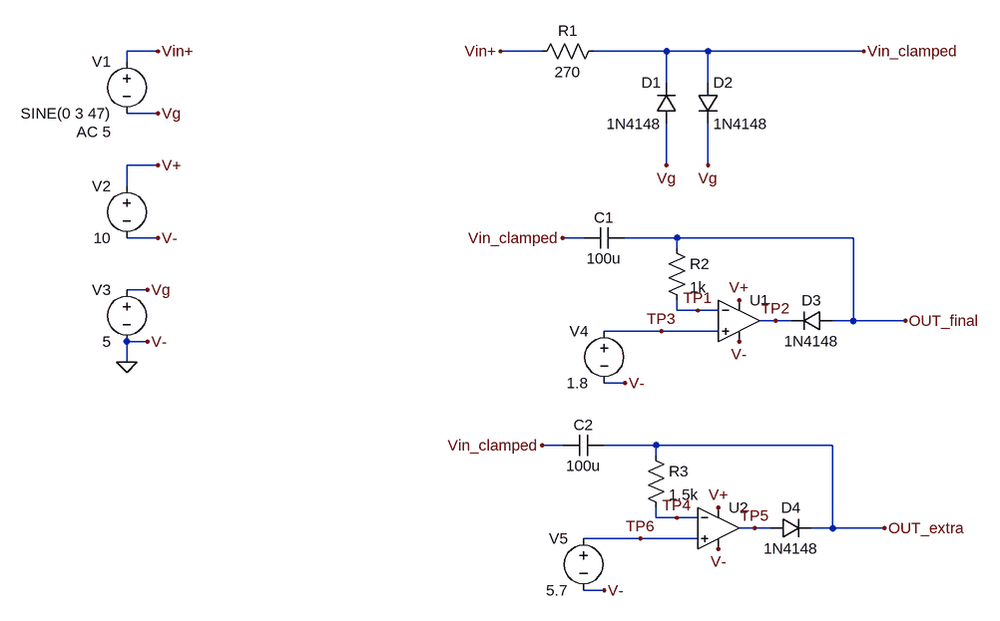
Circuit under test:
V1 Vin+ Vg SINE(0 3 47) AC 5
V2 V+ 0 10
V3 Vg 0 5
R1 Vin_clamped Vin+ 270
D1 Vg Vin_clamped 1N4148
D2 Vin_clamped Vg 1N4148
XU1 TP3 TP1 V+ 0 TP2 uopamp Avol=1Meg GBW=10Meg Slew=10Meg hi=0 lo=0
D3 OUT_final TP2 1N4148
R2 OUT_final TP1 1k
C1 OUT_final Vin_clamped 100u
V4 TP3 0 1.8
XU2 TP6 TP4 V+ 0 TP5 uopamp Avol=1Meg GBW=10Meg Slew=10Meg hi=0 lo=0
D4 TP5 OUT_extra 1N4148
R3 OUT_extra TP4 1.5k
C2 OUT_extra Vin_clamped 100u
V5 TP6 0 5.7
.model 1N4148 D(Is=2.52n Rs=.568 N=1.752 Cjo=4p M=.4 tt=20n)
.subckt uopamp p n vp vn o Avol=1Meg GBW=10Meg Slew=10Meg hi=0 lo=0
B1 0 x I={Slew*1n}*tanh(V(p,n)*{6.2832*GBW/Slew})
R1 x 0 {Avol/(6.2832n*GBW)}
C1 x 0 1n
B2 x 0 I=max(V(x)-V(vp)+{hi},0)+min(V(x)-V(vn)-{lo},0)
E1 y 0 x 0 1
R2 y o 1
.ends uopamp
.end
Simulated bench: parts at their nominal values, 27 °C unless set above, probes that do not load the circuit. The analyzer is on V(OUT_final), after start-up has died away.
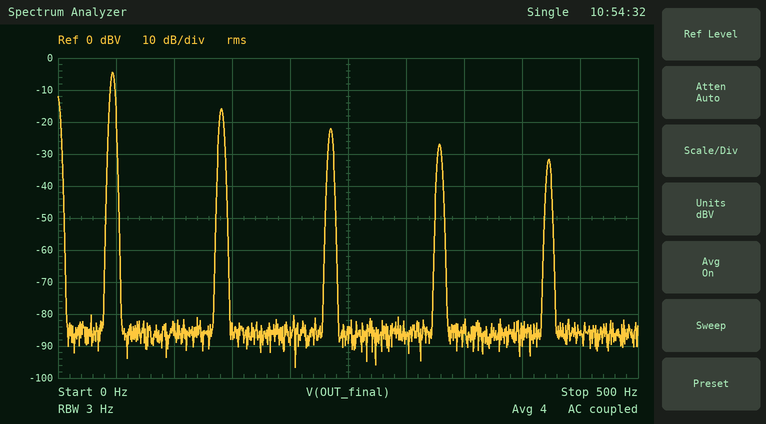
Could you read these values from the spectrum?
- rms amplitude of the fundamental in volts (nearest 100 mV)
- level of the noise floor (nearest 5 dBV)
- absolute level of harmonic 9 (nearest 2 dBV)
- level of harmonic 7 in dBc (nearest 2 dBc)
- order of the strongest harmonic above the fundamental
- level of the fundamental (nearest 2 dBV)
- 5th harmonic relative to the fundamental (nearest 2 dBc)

600 mV
-85 dBV
-32 dBV
-22 dBc
3
-4 dBV
-18 dBc
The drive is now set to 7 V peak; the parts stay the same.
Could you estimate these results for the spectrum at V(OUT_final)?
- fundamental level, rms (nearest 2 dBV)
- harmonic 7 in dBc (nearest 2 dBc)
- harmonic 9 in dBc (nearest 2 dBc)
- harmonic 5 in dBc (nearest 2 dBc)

-4 dBV
-20 dBc
-22 dBc
-16 dBc
